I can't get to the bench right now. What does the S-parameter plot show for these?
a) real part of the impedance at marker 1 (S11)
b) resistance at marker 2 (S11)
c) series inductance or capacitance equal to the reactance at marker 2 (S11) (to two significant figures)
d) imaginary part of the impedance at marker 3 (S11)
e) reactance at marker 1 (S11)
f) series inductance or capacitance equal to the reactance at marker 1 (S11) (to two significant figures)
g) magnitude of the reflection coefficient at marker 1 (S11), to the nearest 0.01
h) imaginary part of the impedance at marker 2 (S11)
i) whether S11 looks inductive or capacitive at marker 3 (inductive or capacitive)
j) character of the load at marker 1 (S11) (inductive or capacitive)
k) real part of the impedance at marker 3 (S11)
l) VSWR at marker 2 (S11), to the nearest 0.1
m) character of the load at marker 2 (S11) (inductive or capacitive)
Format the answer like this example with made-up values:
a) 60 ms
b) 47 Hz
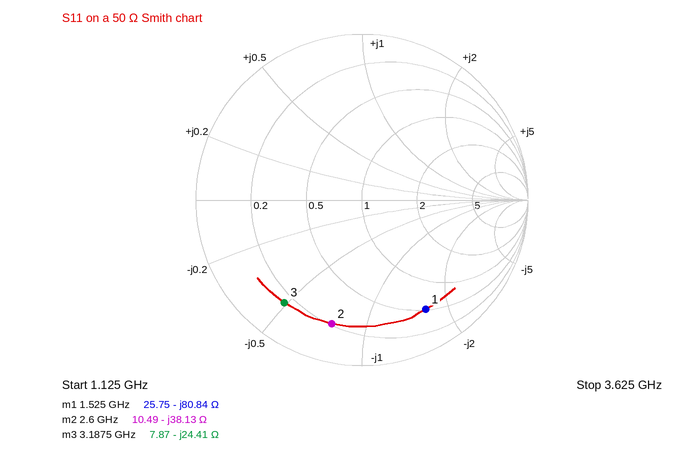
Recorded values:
a) 25.75 Ω
b) 10.49 Ω
c) 1.6 pF
d) -24.41 Ω
e) -80.84 Ω
f) 1.3 pF
g) 0.76
h) -38.13 Ω
i) capacitive
j) capacitive
k) 7.87 Ω
l) 7.6
m) capacitive
